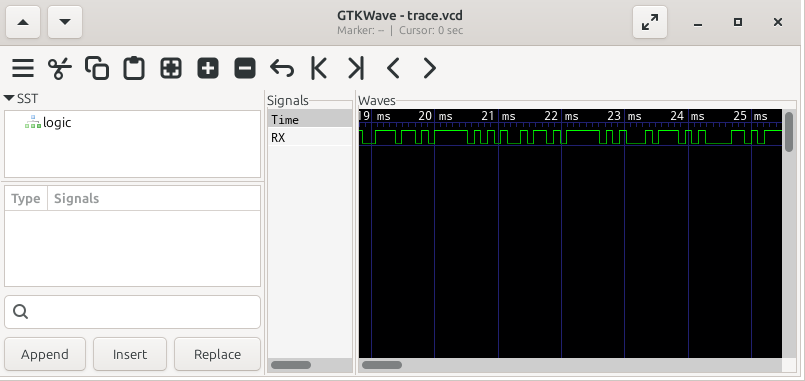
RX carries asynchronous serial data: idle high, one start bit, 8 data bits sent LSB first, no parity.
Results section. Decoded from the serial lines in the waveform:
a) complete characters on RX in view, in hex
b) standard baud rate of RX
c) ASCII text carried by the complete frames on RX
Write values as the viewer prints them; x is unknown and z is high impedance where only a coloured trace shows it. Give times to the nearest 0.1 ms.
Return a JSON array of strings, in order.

["6E, 5F, 69, 5F, 74, 61", "9600 baud", "\"n_i_ta\""]
